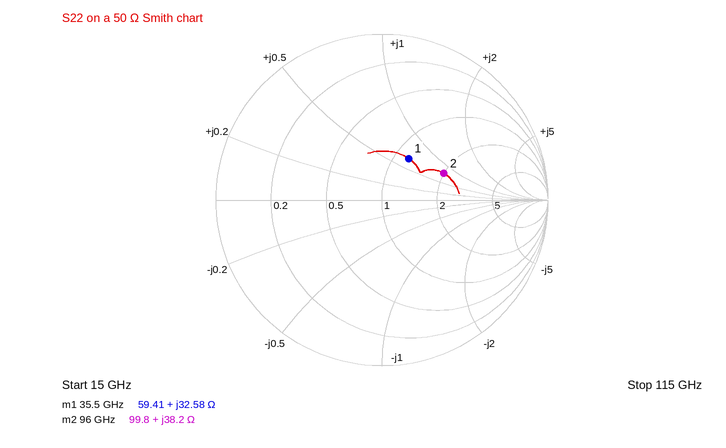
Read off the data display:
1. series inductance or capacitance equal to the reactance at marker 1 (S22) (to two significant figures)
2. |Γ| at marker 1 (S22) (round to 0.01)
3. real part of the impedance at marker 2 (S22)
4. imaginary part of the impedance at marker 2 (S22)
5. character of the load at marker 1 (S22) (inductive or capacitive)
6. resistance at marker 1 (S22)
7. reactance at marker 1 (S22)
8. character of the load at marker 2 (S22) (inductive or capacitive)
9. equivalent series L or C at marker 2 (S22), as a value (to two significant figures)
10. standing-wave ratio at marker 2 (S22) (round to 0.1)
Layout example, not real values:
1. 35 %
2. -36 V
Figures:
1. 150 pH
2. 0.30
3. 99.8 Ω
4. +38.2 Ω
5. inductive
6. 59.41 Ω
7. +32.58 Ω
8. inductive
9. 63 pH
10. 2.4
